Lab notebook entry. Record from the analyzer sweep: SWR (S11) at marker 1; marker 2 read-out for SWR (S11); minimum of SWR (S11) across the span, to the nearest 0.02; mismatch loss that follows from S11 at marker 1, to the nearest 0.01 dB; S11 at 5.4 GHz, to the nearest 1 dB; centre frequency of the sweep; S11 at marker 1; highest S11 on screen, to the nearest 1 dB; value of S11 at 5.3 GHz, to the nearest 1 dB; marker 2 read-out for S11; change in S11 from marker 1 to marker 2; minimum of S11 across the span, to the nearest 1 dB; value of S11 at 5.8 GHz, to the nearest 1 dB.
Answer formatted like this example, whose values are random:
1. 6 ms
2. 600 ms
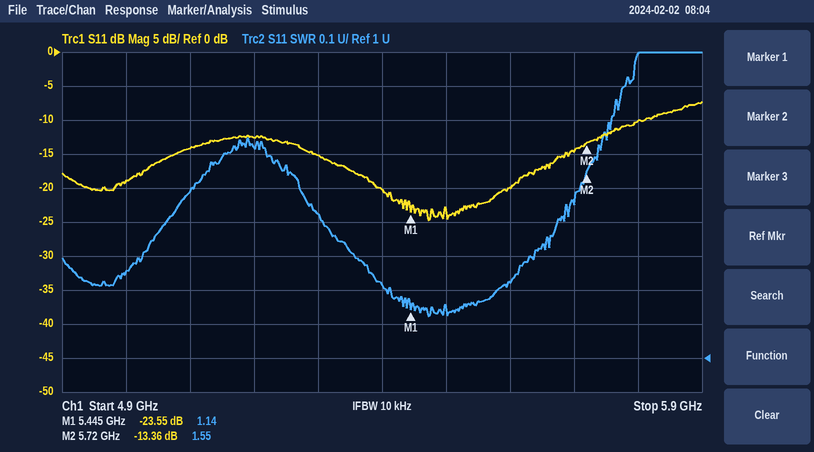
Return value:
1. 1.14
2. 1.55
3. 1.12
4. 0.02 dB
5. -20 dB
6. 5.4 GHz
7. -23.55 dB
8. -7 dB
9. -15 dB
10. -13.36 dB
11. 10.19 dB
12. -25 dB
13. -10 dB
